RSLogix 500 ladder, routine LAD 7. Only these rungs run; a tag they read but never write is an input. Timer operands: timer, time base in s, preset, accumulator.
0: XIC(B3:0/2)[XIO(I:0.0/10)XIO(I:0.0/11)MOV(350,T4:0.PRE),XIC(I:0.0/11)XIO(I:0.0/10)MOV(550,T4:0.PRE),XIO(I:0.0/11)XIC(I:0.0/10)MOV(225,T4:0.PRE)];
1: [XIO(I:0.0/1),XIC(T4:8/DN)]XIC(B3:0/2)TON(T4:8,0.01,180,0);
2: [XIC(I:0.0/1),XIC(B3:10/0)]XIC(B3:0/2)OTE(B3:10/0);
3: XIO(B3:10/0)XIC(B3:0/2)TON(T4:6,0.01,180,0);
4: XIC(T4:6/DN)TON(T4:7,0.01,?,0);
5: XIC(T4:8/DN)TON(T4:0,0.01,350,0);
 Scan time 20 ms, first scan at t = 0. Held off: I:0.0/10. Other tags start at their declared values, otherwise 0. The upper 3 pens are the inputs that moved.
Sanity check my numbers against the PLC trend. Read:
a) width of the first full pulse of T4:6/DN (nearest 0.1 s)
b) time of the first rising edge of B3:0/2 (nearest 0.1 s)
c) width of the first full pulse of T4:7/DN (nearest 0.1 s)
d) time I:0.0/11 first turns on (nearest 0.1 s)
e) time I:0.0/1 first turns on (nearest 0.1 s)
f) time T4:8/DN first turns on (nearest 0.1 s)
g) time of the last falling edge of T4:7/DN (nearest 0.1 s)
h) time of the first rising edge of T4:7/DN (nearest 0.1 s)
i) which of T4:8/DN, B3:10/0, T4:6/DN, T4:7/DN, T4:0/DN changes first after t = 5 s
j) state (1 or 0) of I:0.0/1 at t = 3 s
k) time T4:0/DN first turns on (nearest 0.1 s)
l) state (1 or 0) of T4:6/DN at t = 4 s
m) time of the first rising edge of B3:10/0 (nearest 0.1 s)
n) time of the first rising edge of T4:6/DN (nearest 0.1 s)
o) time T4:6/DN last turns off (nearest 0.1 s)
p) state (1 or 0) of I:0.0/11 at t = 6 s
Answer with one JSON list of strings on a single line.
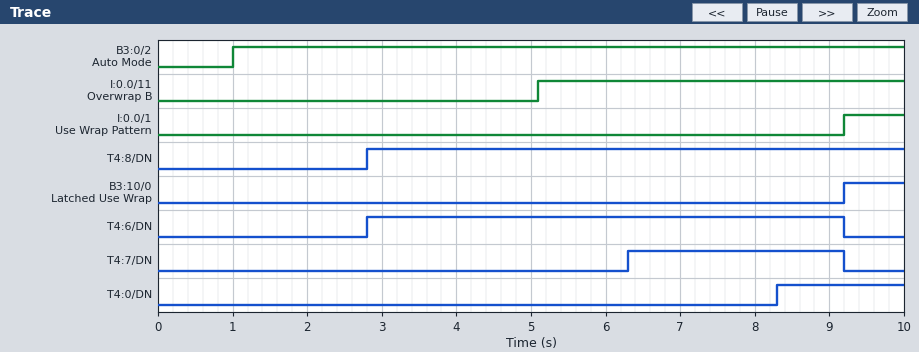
["6.4 s", "1.0 s", "2.9 s", "5.1 s", "9.2 s", "2.8 s", "9.2 s", "6.3 s", "T4:7/DN", "0", "8.3 s", "1", "9.2 s", "2.8 s", "9.2 s", "1"]
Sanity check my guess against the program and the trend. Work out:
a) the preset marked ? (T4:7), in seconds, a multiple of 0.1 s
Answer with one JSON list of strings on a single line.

["3.5 s"]
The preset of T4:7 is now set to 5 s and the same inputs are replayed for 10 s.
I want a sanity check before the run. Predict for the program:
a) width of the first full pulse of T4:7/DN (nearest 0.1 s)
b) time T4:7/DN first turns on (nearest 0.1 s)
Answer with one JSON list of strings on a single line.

["1.4 s", "7.8 s"]
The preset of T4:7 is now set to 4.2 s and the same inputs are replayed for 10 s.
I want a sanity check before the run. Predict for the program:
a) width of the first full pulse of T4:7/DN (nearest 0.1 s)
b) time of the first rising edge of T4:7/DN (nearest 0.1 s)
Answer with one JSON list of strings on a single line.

["2.2 s", "7.0 s"]
